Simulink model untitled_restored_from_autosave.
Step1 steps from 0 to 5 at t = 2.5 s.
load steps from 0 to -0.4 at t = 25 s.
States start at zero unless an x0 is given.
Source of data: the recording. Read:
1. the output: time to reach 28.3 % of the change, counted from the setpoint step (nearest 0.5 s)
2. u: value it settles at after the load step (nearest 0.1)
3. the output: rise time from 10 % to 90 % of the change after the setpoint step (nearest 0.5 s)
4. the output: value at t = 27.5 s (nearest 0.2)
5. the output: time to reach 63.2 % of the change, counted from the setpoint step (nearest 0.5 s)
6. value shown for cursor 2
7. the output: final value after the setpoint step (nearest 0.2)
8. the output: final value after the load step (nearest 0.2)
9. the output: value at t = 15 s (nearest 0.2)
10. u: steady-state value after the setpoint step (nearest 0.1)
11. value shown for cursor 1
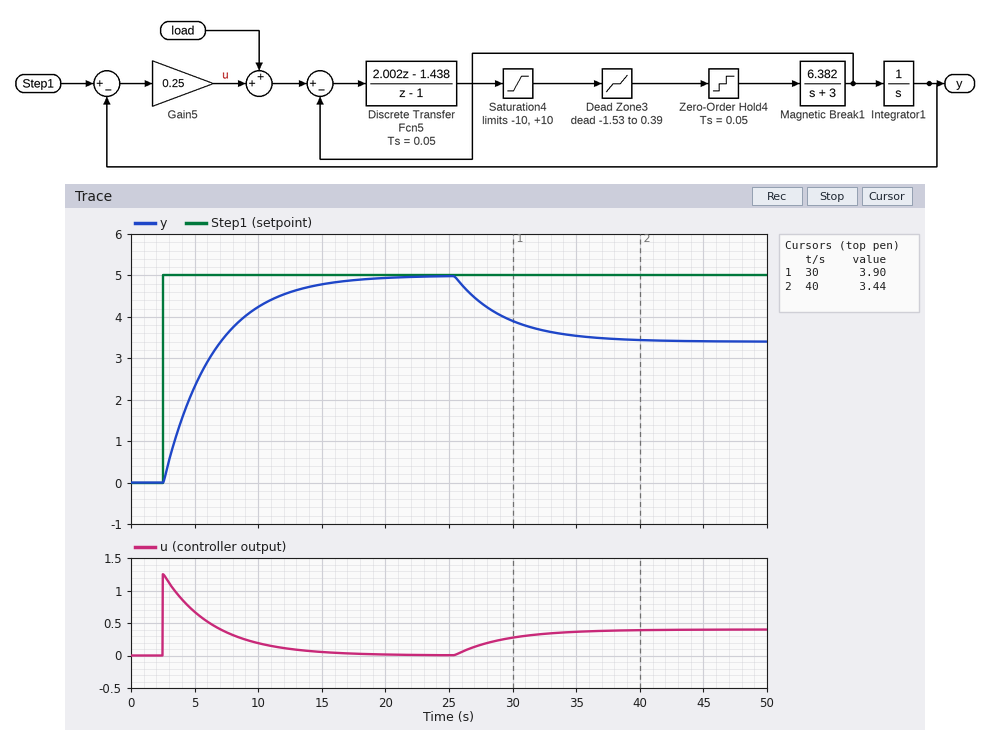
1.5 s
0.4
8.5 s
4.4
4.0 s
3.44
5.0
3.4
4.8
0.0
3.90
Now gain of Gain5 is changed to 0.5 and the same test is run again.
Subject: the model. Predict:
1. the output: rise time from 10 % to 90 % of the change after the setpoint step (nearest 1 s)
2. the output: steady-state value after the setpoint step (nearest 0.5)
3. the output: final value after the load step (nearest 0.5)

4 s
5.0
4.0
